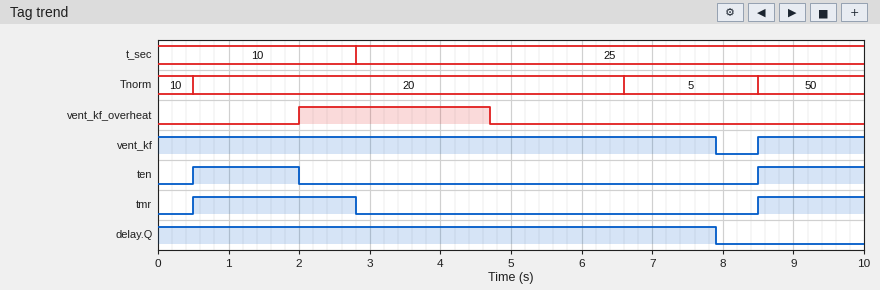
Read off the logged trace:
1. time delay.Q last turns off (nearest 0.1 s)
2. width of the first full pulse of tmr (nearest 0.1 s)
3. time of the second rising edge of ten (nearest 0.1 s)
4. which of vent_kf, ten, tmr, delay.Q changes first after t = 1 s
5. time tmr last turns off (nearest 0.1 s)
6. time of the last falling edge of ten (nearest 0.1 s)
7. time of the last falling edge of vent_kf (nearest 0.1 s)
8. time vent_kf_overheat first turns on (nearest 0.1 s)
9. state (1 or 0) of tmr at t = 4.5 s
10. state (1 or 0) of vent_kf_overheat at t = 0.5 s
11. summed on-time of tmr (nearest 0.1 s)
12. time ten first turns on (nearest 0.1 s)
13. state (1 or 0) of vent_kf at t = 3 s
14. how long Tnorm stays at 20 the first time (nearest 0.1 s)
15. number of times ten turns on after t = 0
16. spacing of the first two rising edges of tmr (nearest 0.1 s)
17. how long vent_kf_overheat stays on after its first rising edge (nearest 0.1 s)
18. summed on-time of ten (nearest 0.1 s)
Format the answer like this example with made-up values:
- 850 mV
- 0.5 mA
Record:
- 7.9 s
- 2.3 s
- 8.5 s
- ten
- 2.8 s
- 2.0 s
- 7.9 s
- 2.0 s
- 0
- 0
- 3.8 s
- 0.5 s
- 1
- 6.1 s
- 2
- 8.0 s
- 2.7 s
- 3.0 s
